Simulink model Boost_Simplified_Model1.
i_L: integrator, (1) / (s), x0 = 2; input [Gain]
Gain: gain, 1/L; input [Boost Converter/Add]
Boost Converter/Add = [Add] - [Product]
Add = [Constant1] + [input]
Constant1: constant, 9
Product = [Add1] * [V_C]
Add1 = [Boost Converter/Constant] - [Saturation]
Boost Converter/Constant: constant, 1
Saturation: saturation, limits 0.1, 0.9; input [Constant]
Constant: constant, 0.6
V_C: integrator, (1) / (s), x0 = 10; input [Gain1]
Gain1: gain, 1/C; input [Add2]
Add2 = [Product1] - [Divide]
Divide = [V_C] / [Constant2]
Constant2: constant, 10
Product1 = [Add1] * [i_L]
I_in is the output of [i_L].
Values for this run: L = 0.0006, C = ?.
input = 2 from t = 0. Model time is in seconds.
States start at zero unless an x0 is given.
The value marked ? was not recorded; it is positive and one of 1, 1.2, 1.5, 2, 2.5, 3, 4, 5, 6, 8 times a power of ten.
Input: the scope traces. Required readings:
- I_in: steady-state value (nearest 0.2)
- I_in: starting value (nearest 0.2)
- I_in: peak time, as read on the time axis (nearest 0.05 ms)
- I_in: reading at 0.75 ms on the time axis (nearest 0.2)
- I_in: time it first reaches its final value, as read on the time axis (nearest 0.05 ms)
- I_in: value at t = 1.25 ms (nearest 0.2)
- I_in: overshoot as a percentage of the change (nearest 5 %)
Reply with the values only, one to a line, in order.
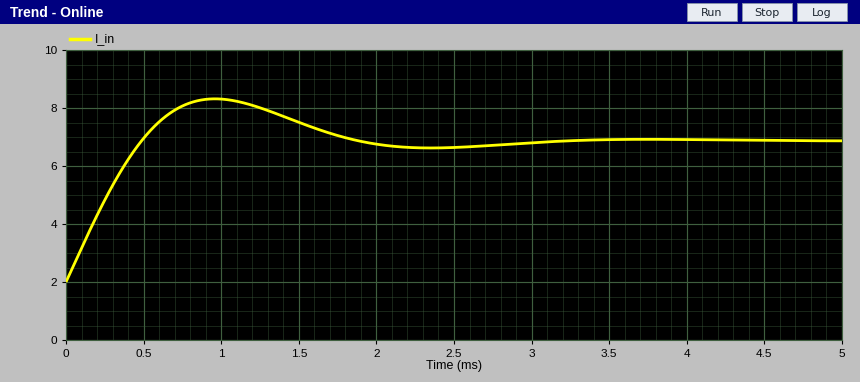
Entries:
6.8
2.0
0.95 ms
8.0
0.50 ms
8.0
30 %
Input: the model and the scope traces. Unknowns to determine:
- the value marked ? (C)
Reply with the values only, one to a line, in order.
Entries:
4e-05
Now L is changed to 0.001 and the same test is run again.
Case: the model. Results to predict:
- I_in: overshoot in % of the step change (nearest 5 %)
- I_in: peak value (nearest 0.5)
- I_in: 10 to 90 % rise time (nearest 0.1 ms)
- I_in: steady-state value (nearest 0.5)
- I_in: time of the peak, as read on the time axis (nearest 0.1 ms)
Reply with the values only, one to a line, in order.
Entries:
10 %
7.5
0.7 ms
7.0
1.5 ms
